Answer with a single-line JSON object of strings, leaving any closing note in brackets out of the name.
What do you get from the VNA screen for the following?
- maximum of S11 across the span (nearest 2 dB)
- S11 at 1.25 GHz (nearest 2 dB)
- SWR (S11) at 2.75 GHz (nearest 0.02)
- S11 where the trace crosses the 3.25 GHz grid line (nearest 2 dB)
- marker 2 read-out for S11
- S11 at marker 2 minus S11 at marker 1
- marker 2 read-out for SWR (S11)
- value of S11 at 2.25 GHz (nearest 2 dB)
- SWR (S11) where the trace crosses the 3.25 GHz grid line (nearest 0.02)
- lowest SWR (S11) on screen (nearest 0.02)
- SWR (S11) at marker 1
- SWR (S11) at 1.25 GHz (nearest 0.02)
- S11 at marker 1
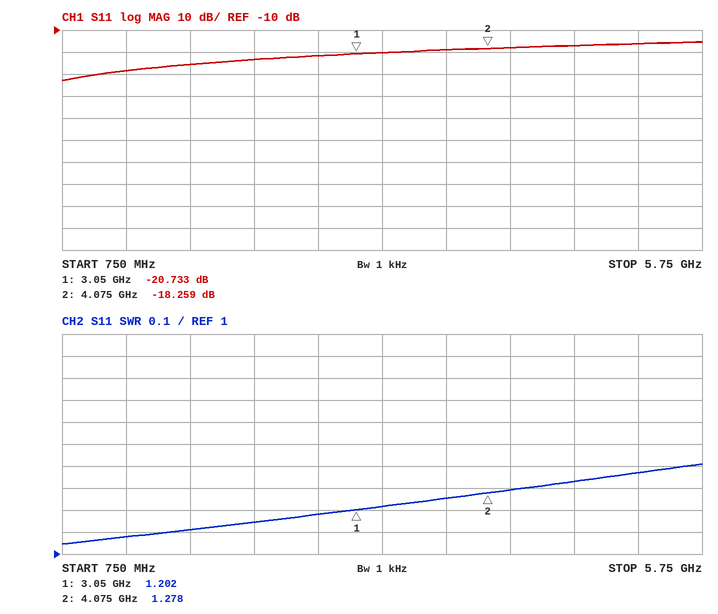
{"maximum of S11 across the span": "-16 dB", "S11 at 1.25 GHz": "-28 dB", "SWR (S11) at 2.75 GHz": "1.18", "S11 where the trace crosses the 3.25 GHz grid line": "-20 dB", "marker 2 read-out for S11": "-18.259 dB", "S11 at marker 2 minus S11 at marker 1": "2.474 dB", "marker 2 read-out for SWR": "1.278", "value of S11 at 2.25 GHz": "-24 dB", "SWR (S11) where the trace crosses the 3.25 GHz grid line": "1.22", "lowest SWR (S11) on screen": "1.04", "SWR (S11) at marker 1": "1.202", "SWR (S11) at 1.25 GHz": "1.08", "S11 at marker 1": "-20.733 dB"}
